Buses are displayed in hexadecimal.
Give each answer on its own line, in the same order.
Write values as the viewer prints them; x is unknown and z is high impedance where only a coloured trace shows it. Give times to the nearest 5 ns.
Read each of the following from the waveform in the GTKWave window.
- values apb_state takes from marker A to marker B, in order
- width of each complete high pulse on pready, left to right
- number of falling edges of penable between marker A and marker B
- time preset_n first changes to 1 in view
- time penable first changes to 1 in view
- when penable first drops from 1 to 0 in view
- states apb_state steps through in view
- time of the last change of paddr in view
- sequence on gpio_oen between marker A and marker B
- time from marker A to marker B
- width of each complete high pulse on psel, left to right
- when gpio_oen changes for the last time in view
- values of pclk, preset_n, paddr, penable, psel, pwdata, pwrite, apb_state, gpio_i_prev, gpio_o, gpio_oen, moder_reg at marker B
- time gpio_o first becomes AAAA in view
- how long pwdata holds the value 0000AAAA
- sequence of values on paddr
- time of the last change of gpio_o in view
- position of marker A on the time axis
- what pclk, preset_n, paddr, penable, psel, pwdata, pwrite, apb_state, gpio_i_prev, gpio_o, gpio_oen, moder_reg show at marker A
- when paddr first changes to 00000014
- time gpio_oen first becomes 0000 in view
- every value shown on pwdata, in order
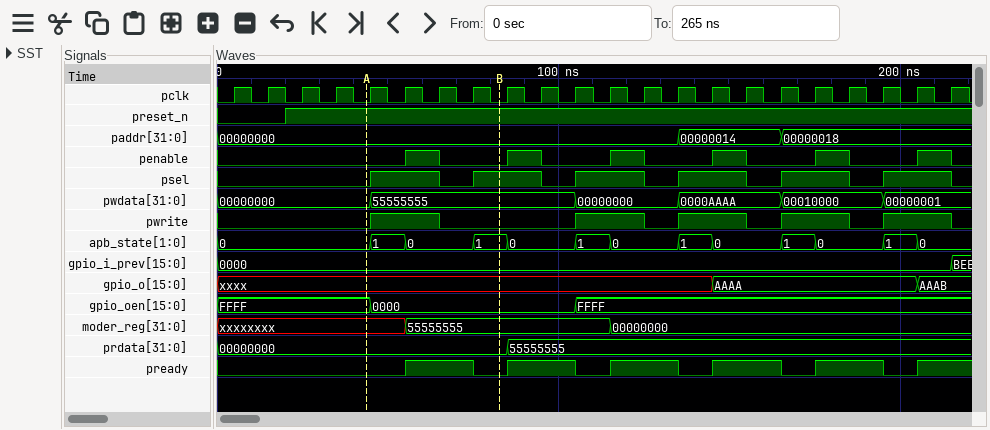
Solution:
0, 1, 0, 1
20 ns, 20 ns, 20 ns, 20 ns, 20 ns
1
20 ns
55 ns
65 ns
0, 1, 0, 1, 0, 1, 0, 1, 0, 1, 0, 1, 0
165 ns
FFFF, 0000
40 ns
20 ns, 20 ns, 20 ns, 20 ns, 20 ns, 20 ns
105 ns
pclk=0, preset_n=1, paddr=00000000, penable=0, psel=1, pwdata=55555555, pwrite=0, apb_state=1, gpio_i_prev=0000, gpio_o=xxxx, gpio_oen=0000, moder_reg=55555555
145 ns
30 ns
00000000, 00000014, 00000018
205 ns
45 ns
pclk=0, preset_n=1, paddr=00000000, penable=0, psel=0, pwdata=00000000, pwrite=0, apb_state=0, gpio_i_prev=0000, gpio_o=xxxx, gpio_oen=FFFF, moder_reg=xxxxxxxx
135 ns
45 ns
00000000, 55555555, 00000000, 0000AAAA, 00010000, 00000001
